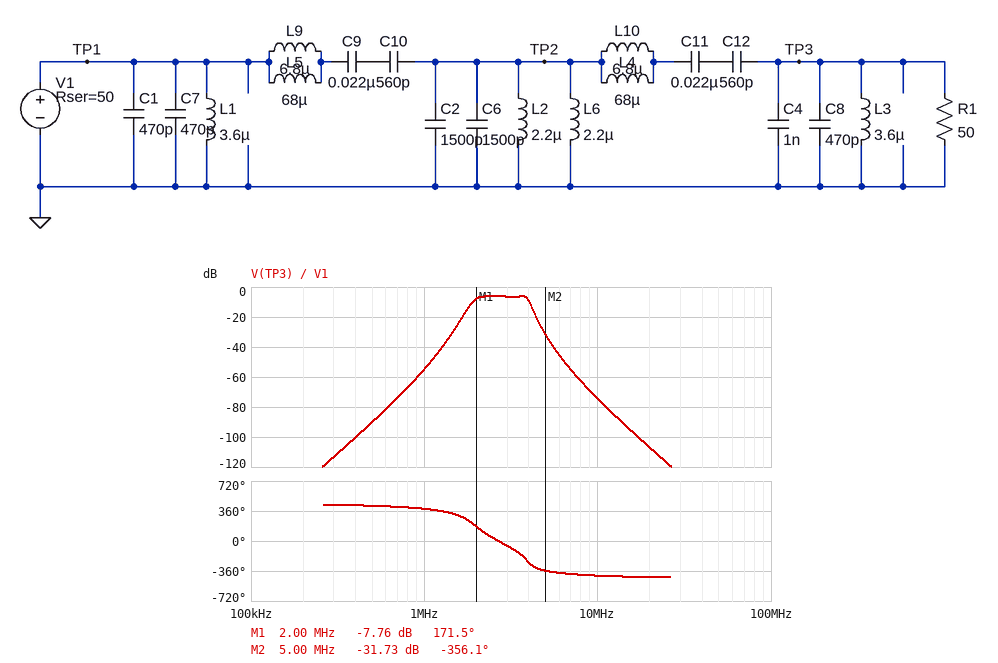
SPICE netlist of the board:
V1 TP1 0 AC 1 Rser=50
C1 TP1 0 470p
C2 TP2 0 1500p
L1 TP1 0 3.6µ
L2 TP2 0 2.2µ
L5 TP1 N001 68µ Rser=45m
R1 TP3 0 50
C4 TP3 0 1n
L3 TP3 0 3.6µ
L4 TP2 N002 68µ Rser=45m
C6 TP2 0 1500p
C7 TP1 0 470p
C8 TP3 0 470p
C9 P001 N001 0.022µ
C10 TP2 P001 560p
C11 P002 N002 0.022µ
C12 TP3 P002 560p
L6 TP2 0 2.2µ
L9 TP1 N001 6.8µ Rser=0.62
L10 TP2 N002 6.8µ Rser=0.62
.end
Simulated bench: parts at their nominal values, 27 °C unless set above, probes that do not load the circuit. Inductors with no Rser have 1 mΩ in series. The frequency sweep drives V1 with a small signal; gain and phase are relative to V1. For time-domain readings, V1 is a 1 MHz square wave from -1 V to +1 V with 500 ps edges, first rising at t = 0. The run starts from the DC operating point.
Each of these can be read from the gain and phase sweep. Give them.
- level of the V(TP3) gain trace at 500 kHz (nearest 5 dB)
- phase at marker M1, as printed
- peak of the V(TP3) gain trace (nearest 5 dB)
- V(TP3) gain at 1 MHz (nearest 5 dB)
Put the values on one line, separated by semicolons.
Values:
-90 dB; 171.5 deg; -5 dB; -55 dB
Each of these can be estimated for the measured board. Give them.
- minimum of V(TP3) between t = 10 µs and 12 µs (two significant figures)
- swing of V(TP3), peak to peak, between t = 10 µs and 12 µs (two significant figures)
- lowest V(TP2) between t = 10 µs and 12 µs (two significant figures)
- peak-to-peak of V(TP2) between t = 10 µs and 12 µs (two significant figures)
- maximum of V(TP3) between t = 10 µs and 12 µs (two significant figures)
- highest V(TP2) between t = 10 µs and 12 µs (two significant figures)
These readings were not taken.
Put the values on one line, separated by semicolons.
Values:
-210 mV; 420 mV; -210 mV; 420 mV; 210 mV; 210 mV
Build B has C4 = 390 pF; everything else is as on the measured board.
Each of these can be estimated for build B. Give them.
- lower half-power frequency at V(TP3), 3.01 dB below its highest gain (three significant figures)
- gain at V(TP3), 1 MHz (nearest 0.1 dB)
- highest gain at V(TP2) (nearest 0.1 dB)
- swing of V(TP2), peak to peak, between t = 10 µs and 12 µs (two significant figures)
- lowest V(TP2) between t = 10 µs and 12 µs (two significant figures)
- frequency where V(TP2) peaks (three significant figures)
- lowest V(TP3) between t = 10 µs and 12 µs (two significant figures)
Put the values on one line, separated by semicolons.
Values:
1.90 MHz; -55.5 dB; -3.7 dB; 520 mV; -260 mV; 3.73 MHz; -220 mV
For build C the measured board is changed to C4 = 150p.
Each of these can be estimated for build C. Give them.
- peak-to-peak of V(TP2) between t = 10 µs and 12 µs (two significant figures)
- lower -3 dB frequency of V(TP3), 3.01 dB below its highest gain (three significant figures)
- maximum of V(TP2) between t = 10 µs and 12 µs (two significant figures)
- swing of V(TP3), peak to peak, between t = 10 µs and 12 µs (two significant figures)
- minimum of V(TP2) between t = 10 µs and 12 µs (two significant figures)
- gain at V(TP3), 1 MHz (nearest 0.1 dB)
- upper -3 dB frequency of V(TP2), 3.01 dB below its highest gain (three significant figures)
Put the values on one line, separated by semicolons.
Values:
550 mV; 1.89 MHz; 270 mV; 430 mV; -270 mV; -55.8 dB; 4.06 MHz
